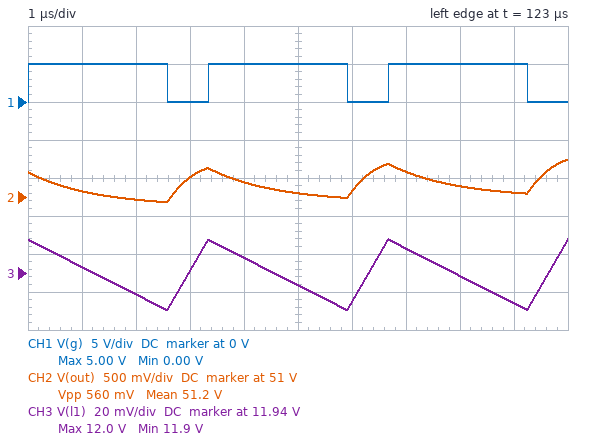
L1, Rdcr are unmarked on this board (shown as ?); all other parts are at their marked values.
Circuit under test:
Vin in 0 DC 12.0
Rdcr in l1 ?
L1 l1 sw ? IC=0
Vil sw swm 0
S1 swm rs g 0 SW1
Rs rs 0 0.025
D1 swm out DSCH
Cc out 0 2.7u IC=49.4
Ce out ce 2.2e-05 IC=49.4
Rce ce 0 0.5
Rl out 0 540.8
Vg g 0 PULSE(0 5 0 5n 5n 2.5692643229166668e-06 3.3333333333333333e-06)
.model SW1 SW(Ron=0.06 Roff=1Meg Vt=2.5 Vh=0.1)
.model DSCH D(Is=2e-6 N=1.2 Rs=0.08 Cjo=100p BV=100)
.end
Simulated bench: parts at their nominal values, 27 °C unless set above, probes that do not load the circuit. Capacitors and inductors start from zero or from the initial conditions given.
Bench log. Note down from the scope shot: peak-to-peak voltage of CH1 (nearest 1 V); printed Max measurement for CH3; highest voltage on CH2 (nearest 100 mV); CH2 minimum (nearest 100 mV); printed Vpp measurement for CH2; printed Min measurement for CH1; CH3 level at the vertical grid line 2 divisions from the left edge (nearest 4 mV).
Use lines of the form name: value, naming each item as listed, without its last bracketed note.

peak-to-peak voltage of CH1: 5 V
printed Max measurement for CH3: 12.0 V
highest voltage on CH2: 51.5 V
CH2 minimum: 50.9 V
printed Vpp measurement for CH2: 560 mV
printed Min measurement for CH1: 0.00 V
CH3 level at the vertical grid line 2 divisions from the left edge: 11.928 V
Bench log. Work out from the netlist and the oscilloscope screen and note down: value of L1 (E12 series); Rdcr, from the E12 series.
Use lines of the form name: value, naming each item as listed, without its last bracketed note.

value of L1: 22 µH
Rdcr, from the E12 series: 0.027 Ω
